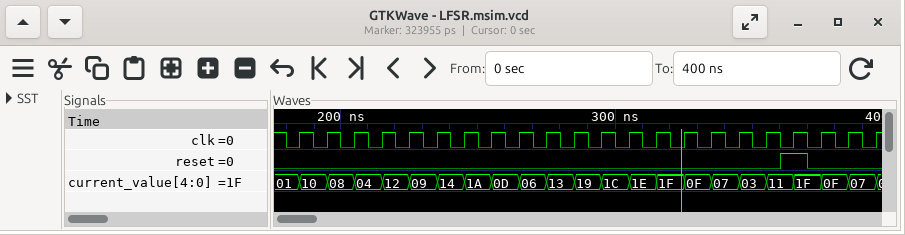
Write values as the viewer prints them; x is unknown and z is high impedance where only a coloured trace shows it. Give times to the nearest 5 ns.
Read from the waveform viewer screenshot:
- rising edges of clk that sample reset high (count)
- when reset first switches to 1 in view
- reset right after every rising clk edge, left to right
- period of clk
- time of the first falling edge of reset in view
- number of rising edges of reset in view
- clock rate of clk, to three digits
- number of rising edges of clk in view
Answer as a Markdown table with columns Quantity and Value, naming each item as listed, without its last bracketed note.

| Quantity | Value |
|---|---|
| rising edges of clk that sample reset high | 1 |
| when reset first switches to 1 in view | 360 ns |
| reset right after every rising clk edge, left to right | 0 0 0 0 0 0 0 0 0 0 0 0 0 0 0 0 0 0 1 0 0 0 |
| period of clk | 10 ns |
| time of the first falling edge of reset in view | 370 ns |
| number of rising edges of reset in view | 1 |
| clock rate of clk, to three digits | 100 MHz |
| number of rising edges of clk in view | 22 |
